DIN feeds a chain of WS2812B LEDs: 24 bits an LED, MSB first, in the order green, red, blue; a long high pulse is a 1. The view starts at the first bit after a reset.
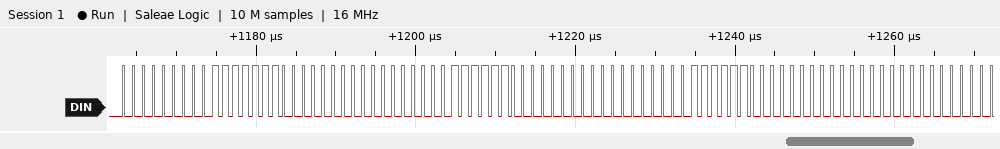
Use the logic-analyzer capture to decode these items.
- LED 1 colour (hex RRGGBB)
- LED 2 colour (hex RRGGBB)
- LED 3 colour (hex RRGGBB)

#7F0000
#7E0000
#7E0000
